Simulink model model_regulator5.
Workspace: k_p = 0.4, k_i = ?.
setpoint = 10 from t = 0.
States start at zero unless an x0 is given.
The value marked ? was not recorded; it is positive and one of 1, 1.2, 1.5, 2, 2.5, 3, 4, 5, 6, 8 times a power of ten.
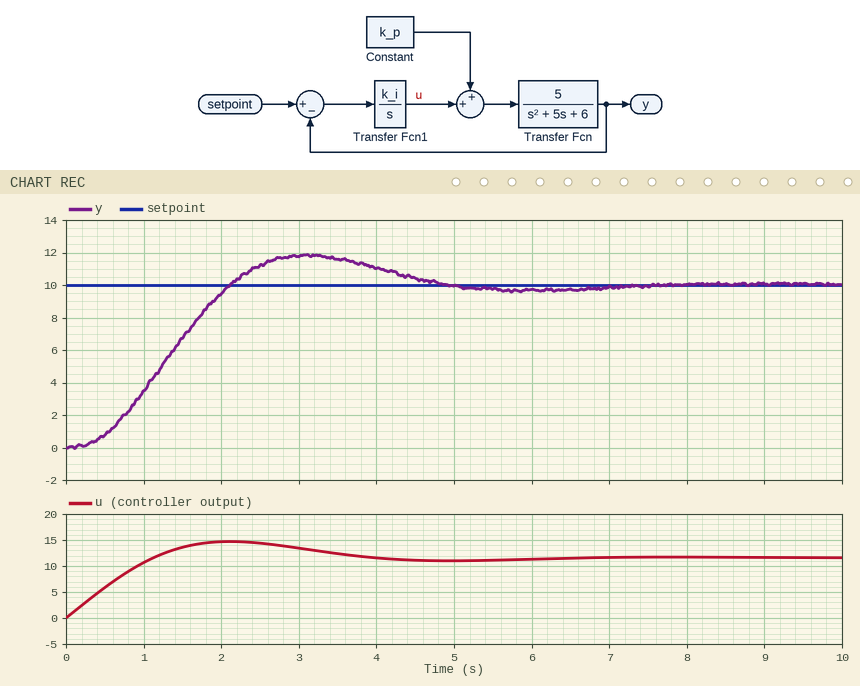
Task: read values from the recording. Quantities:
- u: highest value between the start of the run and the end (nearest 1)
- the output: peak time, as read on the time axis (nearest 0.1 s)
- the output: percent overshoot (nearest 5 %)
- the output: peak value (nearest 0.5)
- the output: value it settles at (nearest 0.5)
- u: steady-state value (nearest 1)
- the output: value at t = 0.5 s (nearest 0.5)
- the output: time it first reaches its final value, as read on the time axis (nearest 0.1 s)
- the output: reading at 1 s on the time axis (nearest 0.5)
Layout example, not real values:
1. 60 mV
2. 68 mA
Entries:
1. 15
2. 3.1 s
3. 20 %
4. 12.0
5. 10.0
6. 12
7. 1.0
8. 2.1 s
9. 3.5
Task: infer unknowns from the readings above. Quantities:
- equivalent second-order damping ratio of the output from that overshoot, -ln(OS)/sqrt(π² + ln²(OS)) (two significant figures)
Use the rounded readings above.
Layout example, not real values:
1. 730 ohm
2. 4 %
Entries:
1. 0.46
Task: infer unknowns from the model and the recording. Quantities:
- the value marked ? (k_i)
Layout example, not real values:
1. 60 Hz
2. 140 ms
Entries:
1. 1.2
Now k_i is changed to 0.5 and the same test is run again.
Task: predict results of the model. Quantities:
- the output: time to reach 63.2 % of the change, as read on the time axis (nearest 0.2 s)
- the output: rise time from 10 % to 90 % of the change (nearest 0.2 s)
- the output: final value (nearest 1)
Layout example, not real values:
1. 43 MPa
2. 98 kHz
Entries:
1. 2.6 s
2. 3.4 s
3. 10
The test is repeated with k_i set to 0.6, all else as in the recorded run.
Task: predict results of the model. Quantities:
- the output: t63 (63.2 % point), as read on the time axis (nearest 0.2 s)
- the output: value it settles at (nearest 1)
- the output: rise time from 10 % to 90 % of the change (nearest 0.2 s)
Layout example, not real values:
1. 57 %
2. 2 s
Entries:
1. 2.2 s
2. 10
3. 2.8 s
